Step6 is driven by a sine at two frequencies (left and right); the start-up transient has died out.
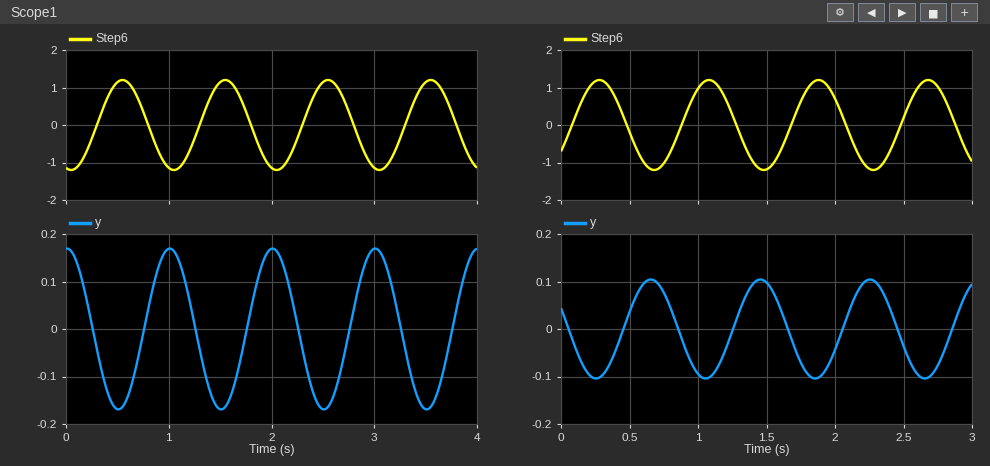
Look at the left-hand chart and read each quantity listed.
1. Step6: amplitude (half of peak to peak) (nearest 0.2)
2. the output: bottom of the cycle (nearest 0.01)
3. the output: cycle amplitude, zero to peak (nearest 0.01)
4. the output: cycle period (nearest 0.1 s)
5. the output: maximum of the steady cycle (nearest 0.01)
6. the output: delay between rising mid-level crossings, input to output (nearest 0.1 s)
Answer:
1.2
-0.17
0.17
1.0 s
0.17
0.5 s
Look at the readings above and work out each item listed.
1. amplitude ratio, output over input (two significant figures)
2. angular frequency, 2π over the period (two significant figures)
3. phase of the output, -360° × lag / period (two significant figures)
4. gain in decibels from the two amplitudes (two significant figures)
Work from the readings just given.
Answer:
0.14
6.3 rad/s
-180°
-17 dB
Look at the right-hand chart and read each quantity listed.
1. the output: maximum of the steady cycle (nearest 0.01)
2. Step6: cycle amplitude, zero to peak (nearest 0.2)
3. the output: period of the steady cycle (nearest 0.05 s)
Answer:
0.10
1.2
0.80 s
